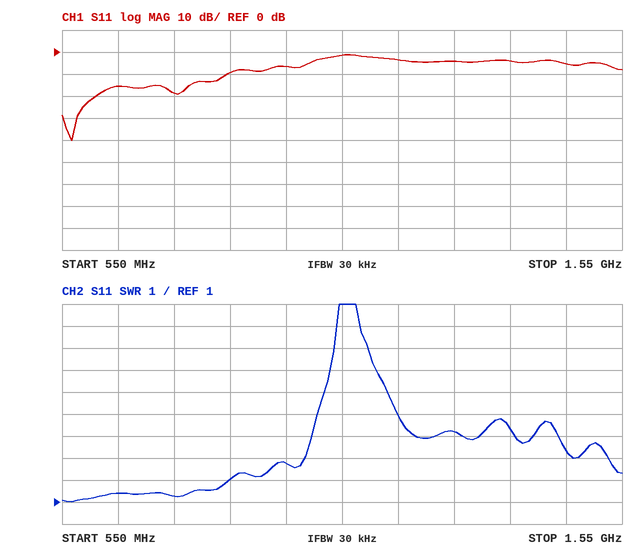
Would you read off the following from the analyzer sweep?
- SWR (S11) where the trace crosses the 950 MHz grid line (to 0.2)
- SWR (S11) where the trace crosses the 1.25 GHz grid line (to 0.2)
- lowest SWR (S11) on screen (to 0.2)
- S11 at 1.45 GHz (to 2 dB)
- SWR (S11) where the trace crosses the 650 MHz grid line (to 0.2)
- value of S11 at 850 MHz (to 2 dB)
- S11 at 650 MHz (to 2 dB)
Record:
2.8
4.2
1.0
-6 dB
1.4
-10 dB
-16 dB
